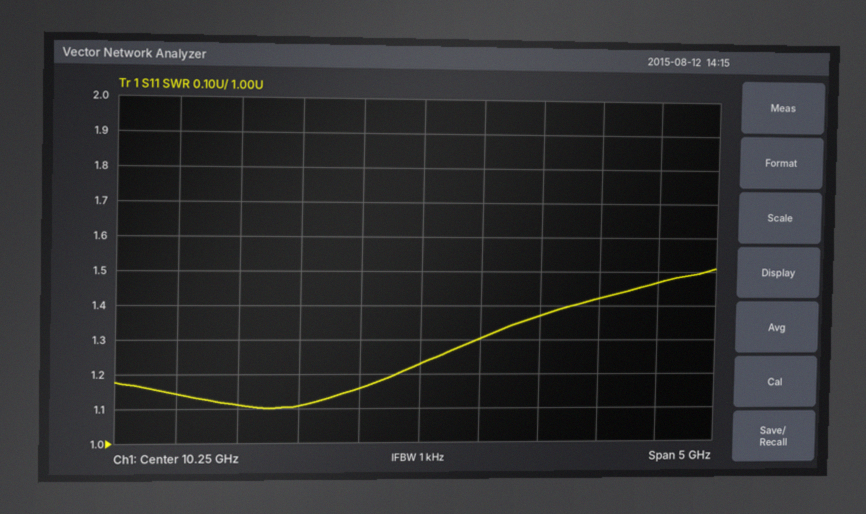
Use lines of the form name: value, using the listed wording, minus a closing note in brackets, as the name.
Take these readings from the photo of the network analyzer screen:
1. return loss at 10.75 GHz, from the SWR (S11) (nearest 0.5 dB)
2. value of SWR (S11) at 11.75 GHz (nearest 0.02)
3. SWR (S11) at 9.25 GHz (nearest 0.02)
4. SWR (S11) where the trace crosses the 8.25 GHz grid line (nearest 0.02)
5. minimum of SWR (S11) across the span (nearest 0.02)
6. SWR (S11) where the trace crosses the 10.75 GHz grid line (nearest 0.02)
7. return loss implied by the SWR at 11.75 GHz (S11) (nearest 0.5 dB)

return loss at 10.75 GHz, from the SWR (S11): 17.5 dB
value of SWR (S11) at 11.75 GHz: 1.42
SWR (S11) at 9.25 GHz: 1.10
SWR (S11) where the trace crosses the 8.25 GHz grid line: 1.14
minimum of SWR (S11) across the span: 1.10
SWR (S11) where the trace crosses the 10.75 GHz grid line: 1.30
return loss implied by the SWR at 11.75 GHz (S11): 15.0 dB
